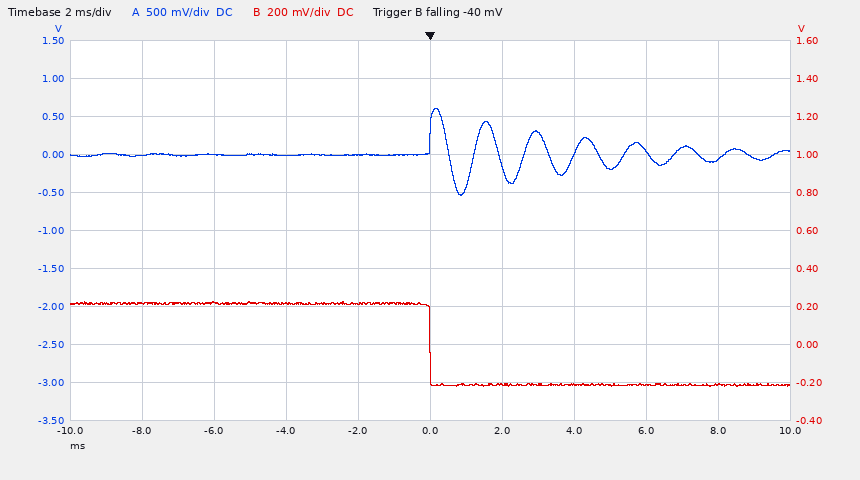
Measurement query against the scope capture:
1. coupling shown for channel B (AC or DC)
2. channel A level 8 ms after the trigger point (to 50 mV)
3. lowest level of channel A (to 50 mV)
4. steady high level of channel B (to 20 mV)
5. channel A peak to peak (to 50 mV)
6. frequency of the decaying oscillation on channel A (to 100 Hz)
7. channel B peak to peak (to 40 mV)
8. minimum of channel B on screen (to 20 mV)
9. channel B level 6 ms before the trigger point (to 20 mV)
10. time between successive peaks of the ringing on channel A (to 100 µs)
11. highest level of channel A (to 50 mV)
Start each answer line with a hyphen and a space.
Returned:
- DC
- -50 mV
- -550 mV
- 220 mV
- 1.15 V
- 700 Hz
- 440 mV
- -220 mV
- 220 mV
- 1.4 ms
- 600 mV
